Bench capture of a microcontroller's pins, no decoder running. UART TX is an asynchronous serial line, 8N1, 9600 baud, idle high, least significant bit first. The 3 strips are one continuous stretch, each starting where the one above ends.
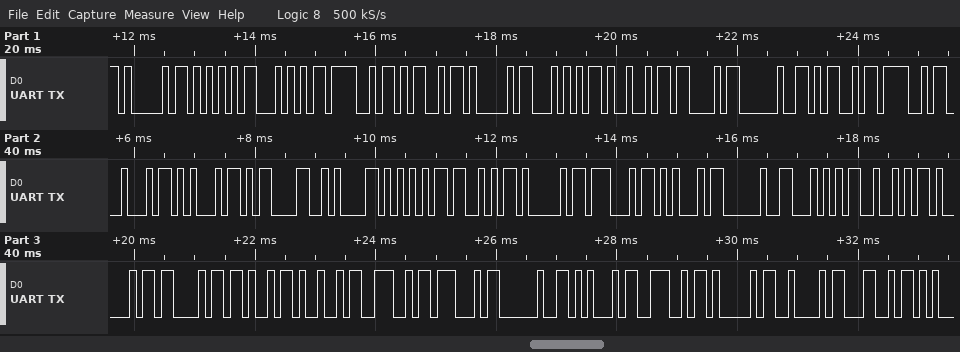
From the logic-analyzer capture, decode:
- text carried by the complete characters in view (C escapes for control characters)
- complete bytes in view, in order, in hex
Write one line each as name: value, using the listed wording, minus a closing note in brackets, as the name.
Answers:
text carried by the complete characters in view: "AUTOMATIC MODE\r\nUSAGE TRACKING ENABL"
complete bytes in view, in order, in hex: 41 55 54 4F 4D 41 54 49 43 20 4D 4F 44 45 0D 0A 55 53 41 47 45 20 54 52 41 43 4B 49 4E 47 20 45 4E 41 42 4C
